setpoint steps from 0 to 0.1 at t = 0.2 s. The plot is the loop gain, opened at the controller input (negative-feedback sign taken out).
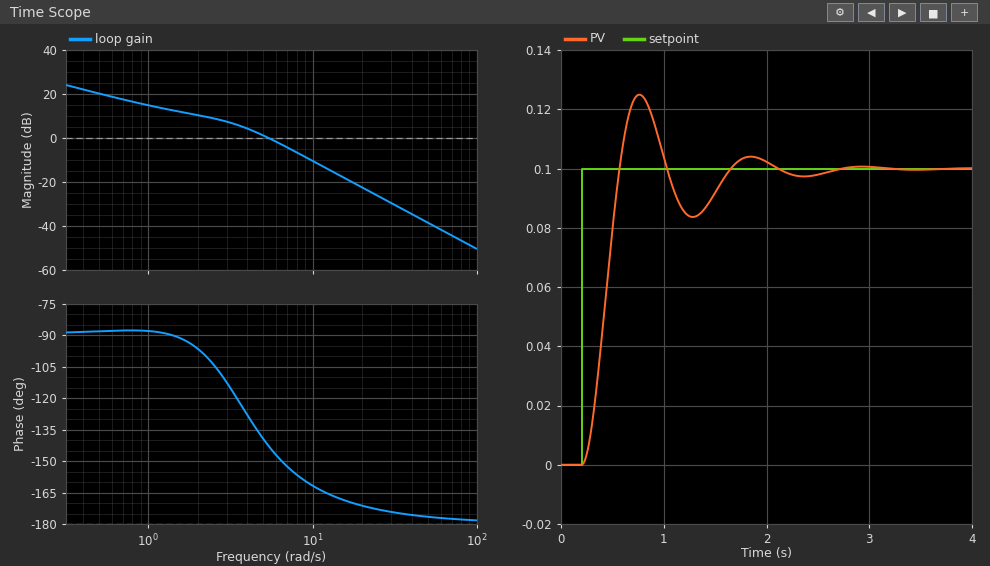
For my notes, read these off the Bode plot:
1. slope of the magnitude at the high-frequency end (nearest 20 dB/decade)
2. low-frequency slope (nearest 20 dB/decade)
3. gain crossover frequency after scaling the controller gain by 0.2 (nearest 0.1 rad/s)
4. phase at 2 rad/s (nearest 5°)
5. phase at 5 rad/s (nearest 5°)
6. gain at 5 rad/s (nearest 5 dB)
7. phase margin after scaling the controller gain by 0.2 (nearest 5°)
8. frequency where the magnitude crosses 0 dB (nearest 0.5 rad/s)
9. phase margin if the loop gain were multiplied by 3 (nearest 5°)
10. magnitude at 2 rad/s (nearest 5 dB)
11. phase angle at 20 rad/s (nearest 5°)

-40 dB/decade
-20 dB/decade
1.1 rad/s
-95°
-140°
0 dB
90°
5.5 rad/s
20°
10 dB
-170°
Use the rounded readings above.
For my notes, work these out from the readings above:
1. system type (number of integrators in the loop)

1
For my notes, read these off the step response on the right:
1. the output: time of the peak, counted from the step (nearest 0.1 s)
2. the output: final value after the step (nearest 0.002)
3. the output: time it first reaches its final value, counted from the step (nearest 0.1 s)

0.6 s
0.100
0.4 s
